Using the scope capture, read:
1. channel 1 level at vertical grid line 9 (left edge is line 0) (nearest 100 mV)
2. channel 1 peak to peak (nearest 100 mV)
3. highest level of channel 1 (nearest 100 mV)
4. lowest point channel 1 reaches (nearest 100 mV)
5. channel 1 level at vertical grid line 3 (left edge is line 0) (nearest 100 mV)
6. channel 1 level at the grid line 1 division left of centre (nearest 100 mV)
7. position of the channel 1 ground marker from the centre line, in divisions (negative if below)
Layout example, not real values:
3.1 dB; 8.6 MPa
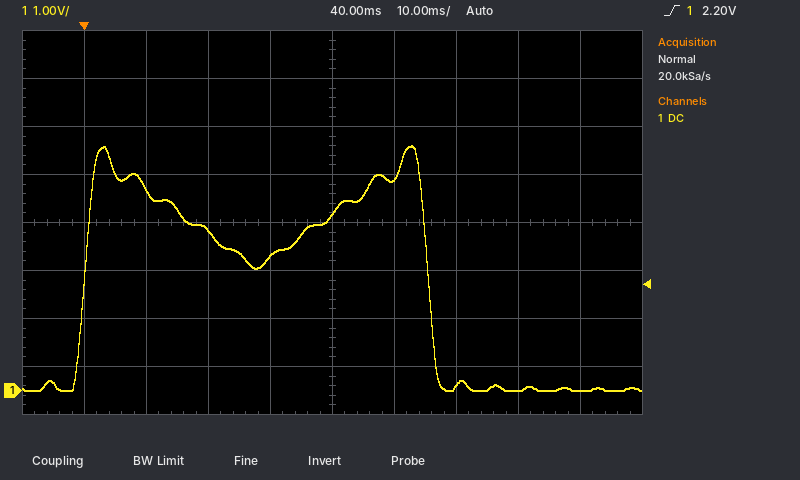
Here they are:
0.0 V; 5.1 V; 5.1 V; 0.0 V; 3.3 V; 2.8 V; -3.5 div
